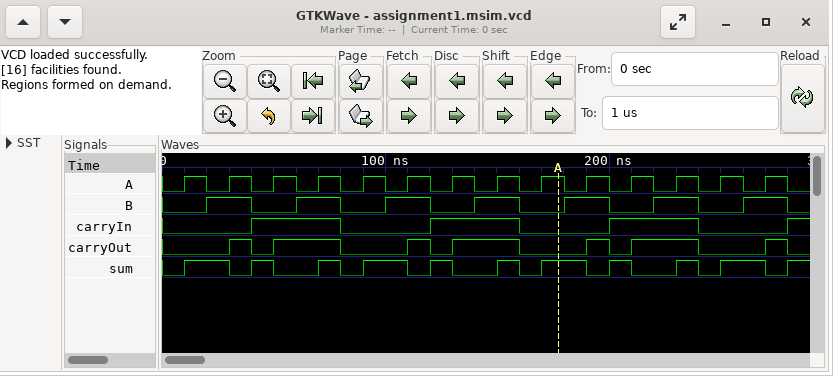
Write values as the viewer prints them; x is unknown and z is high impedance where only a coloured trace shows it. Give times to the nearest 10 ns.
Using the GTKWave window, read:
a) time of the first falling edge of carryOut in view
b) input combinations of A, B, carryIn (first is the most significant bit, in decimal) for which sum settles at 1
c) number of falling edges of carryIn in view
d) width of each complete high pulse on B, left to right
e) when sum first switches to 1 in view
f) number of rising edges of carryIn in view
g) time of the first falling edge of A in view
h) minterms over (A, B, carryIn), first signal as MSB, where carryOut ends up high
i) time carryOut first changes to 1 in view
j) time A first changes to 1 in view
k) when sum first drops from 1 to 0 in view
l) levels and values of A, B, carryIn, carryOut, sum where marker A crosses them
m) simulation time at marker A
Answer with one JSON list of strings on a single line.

["40 ns", "1, 2, 4, 7", "3", "20 ns, 20 ns, 20 ns, 20 ns, 20 ns, 20 ns, 20 ns", "10 ns", "4", "20 ns", "3, 5, 6, 7", "30 ns", "10 ns", "30 ns", "A=1, B=0, carryIn=0, carryOut=0, sum=1", "180 ns"]
